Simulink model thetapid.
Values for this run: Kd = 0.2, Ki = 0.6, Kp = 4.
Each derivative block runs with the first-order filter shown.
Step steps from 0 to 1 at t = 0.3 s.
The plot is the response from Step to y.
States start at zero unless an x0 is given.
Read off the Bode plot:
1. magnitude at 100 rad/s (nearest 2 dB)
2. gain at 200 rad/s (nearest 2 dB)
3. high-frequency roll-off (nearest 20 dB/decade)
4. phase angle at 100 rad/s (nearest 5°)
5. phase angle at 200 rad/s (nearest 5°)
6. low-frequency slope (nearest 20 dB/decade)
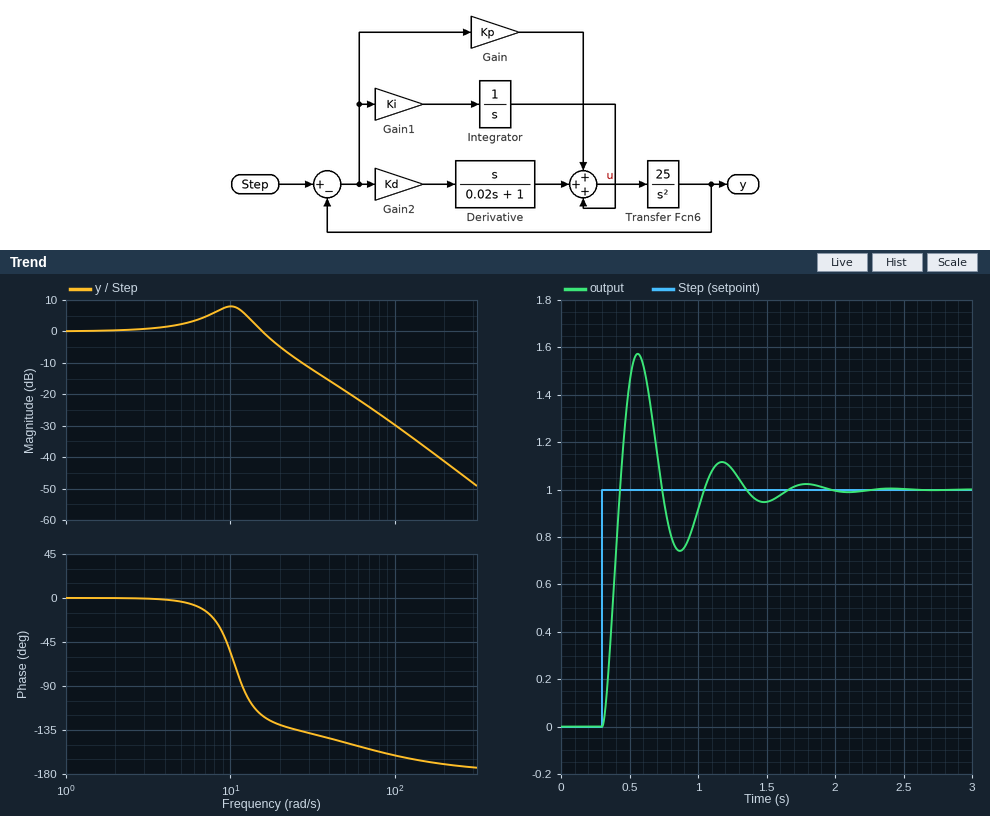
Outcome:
-30 dB
-42 dB
-40 dB/decade
-160°
-170°
0 dB/decade
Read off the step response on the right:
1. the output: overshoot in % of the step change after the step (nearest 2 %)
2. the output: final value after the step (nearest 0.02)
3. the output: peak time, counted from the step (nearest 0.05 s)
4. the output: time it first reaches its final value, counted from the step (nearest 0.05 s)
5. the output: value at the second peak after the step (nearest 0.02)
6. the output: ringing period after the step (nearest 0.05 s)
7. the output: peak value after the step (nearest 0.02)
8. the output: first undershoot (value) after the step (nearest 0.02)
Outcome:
58 %
1.00
0.25 s
0.15 s
1.12
0.60 s
1.58
0.74
